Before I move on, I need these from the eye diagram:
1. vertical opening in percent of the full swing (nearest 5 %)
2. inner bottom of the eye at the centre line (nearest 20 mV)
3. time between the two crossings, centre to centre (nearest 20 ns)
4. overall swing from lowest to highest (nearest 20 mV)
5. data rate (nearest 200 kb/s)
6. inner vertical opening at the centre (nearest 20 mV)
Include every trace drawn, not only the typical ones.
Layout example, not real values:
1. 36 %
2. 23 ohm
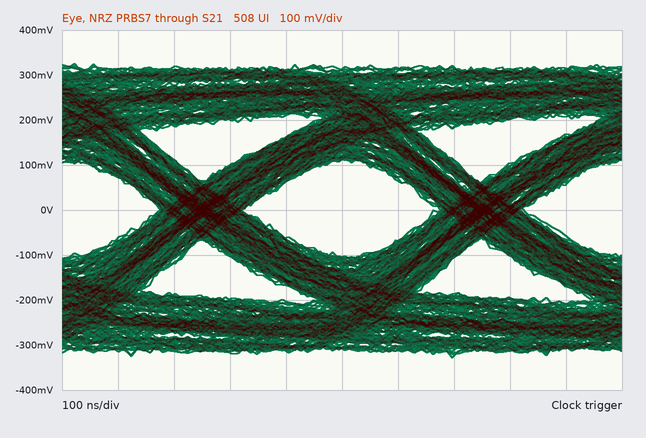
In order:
1. 35 %
2. -100 mV
3. 500 ns
4. 660 mV
5. 2.0 Mb/s
6. 220 mV
